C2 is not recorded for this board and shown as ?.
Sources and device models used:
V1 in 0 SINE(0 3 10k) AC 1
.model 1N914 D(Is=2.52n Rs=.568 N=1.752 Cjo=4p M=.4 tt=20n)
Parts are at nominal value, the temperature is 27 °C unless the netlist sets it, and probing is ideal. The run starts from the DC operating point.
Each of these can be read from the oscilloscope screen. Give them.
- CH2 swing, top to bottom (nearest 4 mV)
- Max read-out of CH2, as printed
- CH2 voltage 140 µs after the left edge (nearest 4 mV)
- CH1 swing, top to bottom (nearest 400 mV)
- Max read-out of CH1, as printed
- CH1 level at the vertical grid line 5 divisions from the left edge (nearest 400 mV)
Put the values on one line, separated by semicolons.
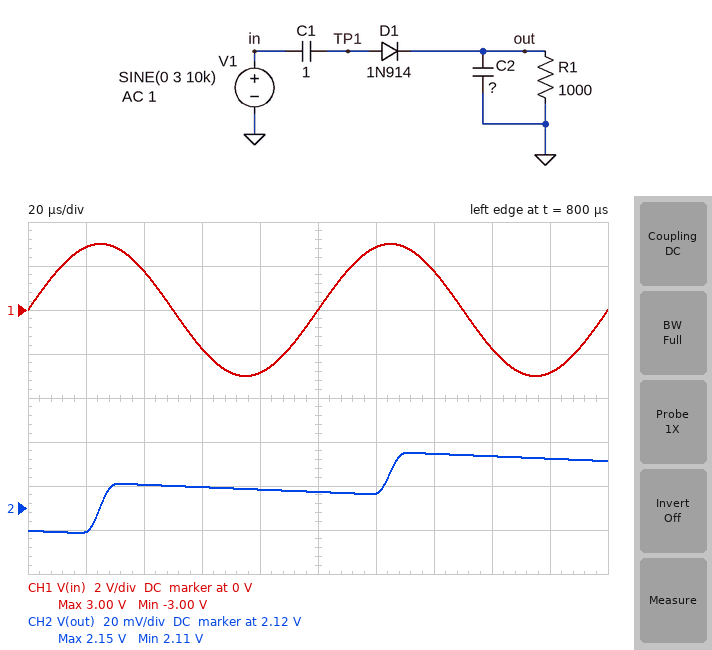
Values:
36 mV; 2.15 V; 2.144 V; 6.0 V; 3.00 V; 0 V
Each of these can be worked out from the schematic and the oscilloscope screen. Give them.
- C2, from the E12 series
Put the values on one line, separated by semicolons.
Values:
39 µF
